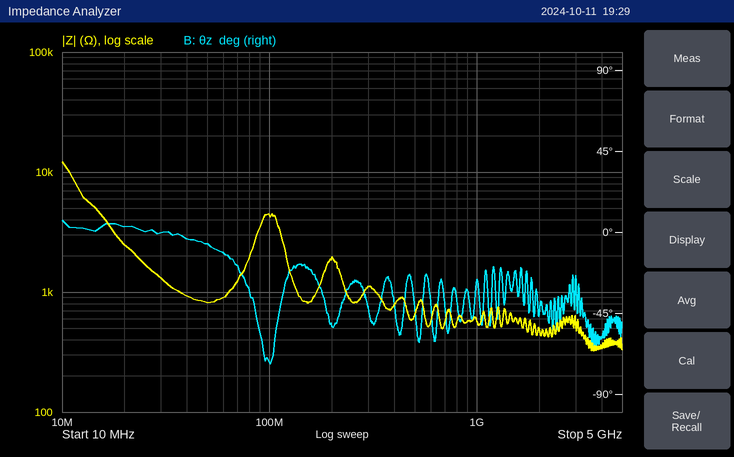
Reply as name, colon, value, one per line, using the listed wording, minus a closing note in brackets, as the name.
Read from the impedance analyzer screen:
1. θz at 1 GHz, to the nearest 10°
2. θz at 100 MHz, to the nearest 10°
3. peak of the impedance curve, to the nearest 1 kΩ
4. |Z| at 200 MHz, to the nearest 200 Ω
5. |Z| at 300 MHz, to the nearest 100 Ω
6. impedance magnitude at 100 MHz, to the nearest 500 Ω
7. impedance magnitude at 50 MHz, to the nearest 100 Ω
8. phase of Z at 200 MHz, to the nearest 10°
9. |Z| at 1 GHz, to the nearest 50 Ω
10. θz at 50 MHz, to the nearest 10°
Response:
θz at 1 GHz, to the nearest 10°: -30°
θz at 100 MHz, to the nearest 10°: -70°
peak of the impedance curve, to the nearest 1 kΩ: 12 kΩ
|Z| at 200 MHz, to the nearest 200 Ω: 2.0 kΩ
|Z| at 300 MHz, to the nearest 100 Ω: 1.1 kΩ
impedance magnitude at 100 MHz, to the nearest 500 Ω: 4.5 kΩ
impedance magnitude at 50 MHz, to the nearest 100 Ω: 800 Ω
phase of Z at 200 MHz, to the nearest 10°: -50°
|Z| at 1 GHz, to the nearest 50 Ω: 550 Ω
θz at 50 MHz, to the nearest 10°: -10°
